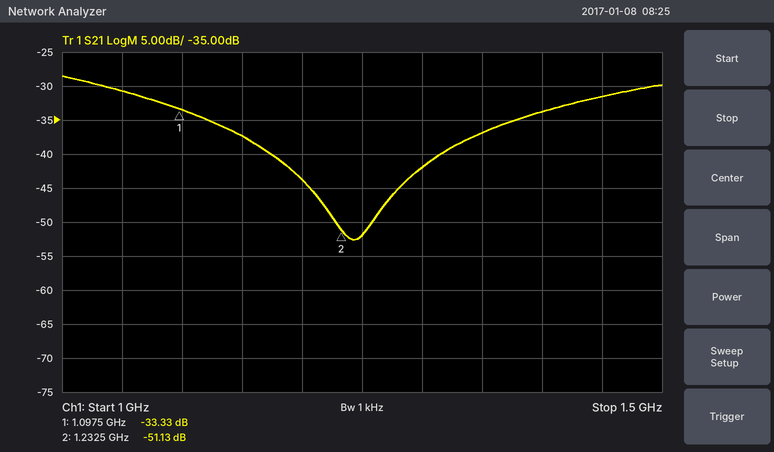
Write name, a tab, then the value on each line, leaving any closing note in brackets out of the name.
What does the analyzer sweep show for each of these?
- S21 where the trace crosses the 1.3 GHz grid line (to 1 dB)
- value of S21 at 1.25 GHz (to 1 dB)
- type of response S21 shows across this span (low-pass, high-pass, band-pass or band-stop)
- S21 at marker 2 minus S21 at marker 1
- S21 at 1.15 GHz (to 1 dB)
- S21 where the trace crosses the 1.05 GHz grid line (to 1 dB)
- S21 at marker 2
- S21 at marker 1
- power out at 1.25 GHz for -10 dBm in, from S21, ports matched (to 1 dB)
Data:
S21 where the trace crosses the 1.3 GHz grid line	-42 dB
value of S21 at 1.25 GHz	-52 dB
type of response S21 shows across this span	band-stop
S21 at marker 2 minus S21 at marker 1	-17.80 dB
S21 at 1.15 GHz	-37 dB
S21 where the trace crosses the 1.05 GHz grid line	-31 dB
S21 at marker 2	-51.13 dB
S21 at marker 1	-33.33 dB
power out at 1.25 GHz for -10 dBm in, from S21, ports matched	-62 dBm
